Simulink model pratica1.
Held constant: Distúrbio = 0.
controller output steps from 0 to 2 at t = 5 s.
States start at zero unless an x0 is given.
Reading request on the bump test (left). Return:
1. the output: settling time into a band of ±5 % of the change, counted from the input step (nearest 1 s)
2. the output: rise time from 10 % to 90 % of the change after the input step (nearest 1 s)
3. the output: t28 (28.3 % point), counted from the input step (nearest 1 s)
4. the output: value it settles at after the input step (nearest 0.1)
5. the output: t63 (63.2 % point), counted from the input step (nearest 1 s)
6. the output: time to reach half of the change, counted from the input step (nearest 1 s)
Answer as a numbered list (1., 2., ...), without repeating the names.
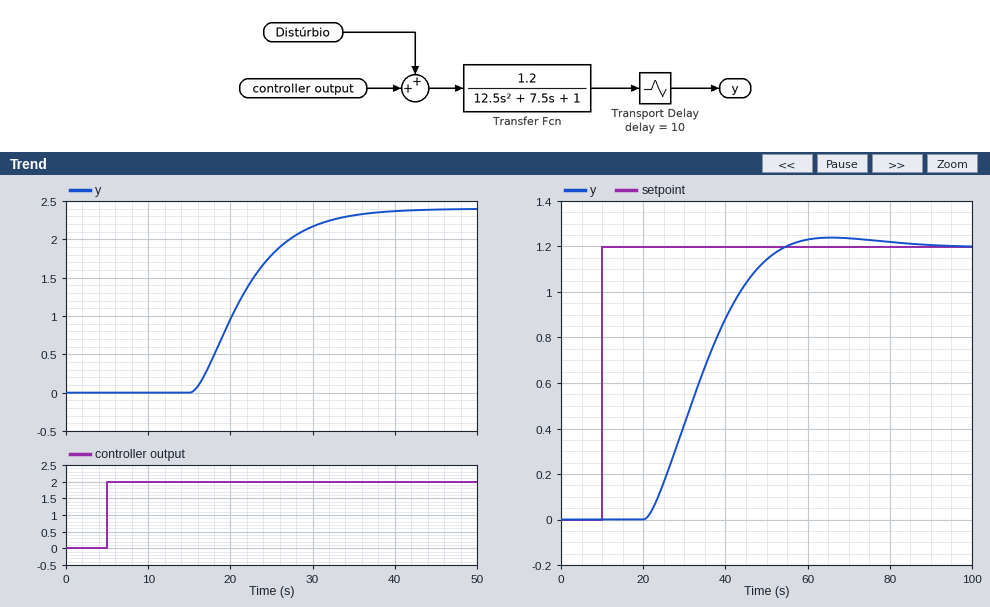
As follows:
1. 28 s
2. 13 s
3. 14 s
4. 2.4
5. 18 s
6. 16 s
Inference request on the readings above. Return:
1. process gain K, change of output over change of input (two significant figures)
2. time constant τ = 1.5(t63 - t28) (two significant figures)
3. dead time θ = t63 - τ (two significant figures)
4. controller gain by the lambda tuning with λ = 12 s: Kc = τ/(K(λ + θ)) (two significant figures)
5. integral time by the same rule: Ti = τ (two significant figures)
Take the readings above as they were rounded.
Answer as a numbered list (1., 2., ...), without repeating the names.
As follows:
1. 1.2
2. 6.0 s
3. 12 s
4. 0.21
5. 6.0 s
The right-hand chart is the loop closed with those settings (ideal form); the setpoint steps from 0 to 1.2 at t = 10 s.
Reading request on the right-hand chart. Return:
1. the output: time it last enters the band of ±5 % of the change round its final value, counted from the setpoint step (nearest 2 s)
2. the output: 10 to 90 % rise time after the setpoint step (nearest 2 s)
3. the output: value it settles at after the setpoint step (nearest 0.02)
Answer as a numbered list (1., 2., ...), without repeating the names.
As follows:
1. 40 s
2. 22 s
3. 1.20
